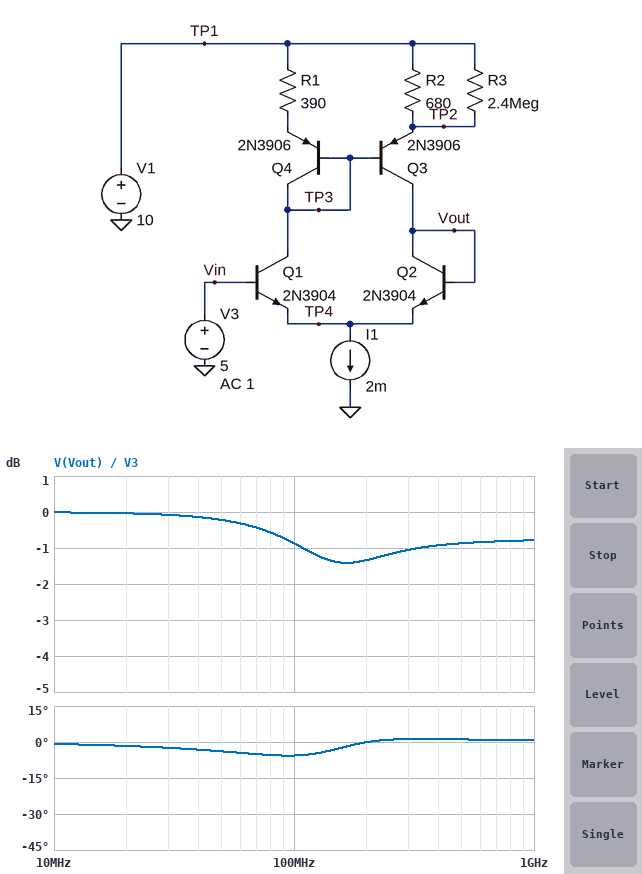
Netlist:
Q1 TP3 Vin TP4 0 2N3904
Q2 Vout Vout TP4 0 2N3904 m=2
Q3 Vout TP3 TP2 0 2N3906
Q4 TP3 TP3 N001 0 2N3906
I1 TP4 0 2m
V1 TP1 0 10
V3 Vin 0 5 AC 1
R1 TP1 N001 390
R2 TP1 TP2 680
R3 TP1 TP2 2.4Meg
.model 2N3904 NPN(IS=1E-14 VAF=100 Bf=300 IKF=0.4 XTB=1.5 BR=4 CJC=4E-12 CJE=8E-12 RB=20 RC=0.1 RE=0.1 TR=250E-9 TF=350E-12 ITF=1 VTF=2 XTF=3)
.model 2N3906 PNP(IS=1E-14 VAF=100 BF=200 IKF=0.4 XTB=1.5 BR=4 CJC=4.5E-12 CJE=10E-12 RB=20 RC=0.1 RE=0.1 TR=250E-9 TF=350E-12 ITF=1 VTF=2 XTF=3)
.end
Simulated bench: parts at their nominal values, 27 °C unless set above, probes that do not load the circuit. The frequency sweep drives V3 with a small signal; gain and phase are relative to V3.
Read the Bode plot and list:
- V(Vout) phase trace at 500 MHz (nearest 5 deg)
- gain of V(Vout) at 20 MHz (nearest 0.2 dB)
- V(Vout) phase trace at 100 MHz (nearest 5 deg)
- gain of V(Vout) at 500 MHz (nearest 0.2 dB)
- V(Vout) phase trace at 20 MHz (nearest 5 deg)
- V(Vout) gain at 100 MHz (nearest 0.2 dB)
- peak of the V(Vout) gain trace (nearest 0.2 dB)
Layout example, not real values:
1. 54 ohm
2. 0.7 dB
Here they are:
1. 0 deg
2. 0 dB
3. -5 deg
4. -0.8 dB
5. 0 deg
6. -0.8 dB
7. 0 dB
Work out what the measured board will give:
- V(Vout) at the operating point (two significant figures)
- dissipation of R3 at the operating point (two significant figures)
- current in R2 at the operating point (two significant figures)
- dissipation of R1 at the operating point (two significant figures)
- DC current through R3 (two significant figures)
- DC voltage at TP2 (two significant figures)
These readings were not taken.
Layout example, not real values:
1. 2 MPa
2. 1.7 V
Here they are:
1. 5.0 V
2. 110 nW
3. 740 µA
4. 610 µW
5. 210 nA
6. 9.5 V
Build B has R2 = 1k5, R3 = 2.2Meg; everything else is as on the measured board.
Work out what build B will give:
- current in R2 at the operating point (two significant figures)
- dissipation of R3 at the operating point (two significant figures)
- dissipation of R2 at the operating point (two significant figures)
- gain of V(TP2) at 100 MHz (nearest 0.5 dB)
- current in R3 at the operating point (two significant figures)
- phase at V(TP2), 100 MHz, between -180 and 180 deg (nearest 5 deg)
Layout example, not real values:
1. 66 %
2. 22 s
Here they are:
1. 430 µA
2. 190 nW
3. 280 µW
4. -5.0 dB
5. 290 nA
6. 70 deg
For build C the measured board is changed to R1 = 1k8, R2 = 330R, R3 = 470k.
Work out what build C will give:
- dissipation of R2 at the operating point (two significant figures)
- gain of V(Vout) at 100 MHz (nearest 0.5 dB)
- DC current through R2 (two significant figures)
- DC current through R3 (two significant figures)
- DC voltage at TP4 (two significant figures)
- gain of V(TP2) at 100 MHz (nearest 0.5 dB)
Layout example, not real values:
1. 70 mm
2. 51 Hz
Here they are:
1. 920 µW
2. -3.5 dB
3. 1.7 mA
4. 1.2 µA
5. 4.4 V
6. 0.5 dB
